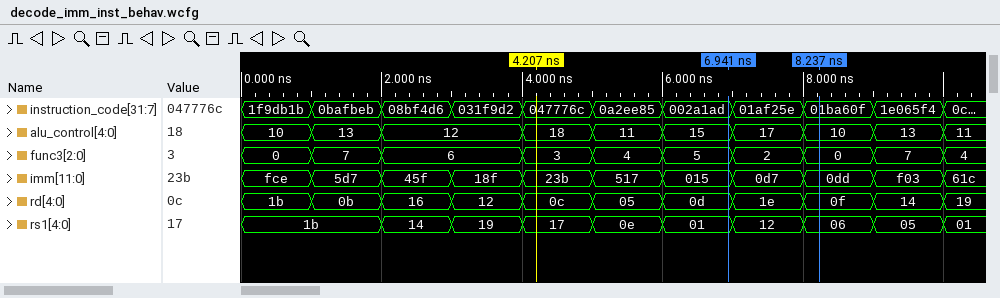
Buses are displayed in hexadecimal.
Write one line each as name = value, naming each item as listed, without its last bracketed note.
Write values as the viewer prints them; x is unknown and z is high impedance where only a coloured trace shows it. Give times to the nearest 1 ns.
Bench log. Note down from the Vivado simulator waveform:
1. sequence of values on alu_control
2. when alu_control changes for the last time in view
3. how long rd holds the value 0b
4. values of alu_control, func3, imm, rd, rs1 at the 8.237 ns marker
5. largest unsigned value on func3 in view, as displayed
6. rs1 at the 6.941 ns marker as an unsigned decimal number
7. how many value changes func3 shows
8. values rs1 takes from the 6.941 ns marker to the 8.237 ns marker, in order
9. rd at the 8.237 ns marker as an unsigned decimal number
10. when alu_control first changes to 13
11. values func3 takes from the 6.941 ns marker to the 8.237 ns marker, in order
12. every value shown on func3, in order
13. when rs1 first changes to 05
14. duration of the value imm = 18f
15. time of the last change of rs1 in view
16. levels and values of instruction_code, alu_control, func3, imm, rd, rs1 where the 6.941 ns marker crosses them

sequence of values on alu_control = 10, 13, 12, 18, 11, 15, 17, 10, 13, 11
when alu_control changes for the last time in view = 10 ns
how long rd holds the value 0b = 1 ns
values of alu_control, func3, imm, rd, rs1 at the 8.237 ns marker = alu_control=10, func3=0, imm=0dd, rd=0f, rs1=06
largest unsigned value on func3 in view, as displayed = 7
rs1 at the 6.941 ns marker as an unsigned decimal number = 1
how many value changes func3 shows = 9
values rs1 takes from the 6.941 ns marker to the 8.237 ns marker, in order = 01, 12, 06
rd at the 8.237 ns marker as an unsigned decimal number = 15
when alu_control first changes to 13 = 1 ns
values func3 takes from the 6.941 ns marker to the 8.237 ns marker, in order = 5, 2, 0
every value shown on func3, in order = 0, 7, 6, 3, 4, 5, 2, 0, 7, 4
when rs1 first changes to 05 = 9 ns
duration of the value imm = 18f = 1 ns
time of the last change of rs1 in view = 10 ns
levels and values of instruction_code, alu_control, func3, imm, rd, rs1 where the 6.941 ns marker crosses them = instruction_code=002a1ad, alu_control=15, func3=5, imm=015, rd=0d, rs1=01
